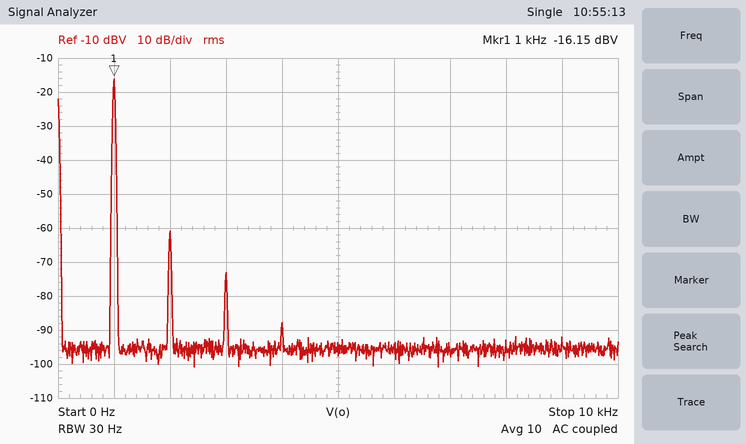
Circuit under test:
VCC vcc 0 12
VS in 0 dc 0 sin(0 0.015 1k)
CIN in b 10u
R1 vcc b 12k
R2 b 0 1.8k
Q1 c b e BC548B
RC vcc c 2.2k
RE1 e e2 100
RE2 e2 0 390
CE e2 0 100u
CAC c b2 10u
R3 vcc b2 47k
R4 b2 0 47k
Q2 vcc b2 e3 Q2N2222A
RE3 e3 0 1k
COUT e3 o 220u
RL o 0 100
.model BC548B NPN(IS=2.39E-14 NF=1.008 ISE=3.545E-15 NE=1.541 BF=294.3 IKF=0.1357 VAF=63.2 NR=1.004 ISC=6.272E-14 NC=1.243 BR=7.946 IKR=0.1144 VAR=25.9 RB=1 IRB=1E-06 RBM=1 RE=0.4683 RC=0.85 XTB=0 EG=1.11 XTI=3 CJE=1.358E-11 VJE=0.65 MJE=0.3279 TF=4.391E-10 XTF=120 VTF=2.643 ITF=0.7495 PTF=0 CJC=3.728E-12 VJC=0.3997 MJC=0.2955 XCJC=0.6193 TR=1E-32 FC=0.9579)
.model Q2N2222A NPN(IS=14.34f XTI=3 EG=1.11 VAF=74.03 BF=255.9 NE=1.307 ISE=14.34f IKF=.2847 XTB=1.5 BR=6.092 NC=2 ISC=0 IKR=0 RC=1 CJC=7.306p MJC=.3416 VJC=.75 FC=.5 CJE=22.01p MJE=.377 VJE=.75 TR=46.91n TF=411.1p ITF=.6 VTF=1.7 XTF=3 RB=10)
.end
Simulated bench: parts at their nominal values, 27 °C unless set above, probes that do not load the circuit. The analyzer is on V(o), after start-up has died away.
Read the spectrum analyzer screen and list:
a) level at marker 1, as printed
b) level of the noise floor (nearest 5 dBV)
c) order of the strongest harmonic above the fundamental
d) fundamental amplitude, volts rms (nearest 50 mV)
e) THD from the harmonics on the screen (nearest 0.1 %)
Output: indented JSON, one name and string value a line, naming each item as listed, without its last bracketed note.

{
  "level at marker 1, as printed": "-16.15 dBV",
  "level of the noise floor": "-95 dBV",
  "order of the strongest harmonic above the fundamental": "2",
  "fundamental amplitude, volts rms": "150 mV",
  "THD from the harmonics on the screen": "0.6 %"
}
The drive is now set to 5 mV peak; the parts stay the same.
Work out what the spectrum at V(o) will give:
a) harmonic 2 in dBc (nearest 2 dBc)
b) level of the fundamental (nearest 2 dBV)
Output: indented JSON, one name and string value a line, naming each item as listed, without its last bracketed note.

{
  "harmonic 2 in dBc": "-56 dBc",
  "level of the fundamental": "-26 dBV"
}
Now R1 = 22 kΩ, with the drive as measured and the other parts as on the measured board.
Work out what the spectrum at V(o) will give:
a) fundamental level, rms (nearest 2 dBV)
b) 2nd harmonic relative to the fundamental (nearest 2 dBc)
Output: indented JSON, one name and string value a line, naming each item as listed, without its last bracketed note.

{
  "fundamental level, rms": "-18 dBV",
  "2nd harmonic relative to the fundamental": "-42 dBc"
}
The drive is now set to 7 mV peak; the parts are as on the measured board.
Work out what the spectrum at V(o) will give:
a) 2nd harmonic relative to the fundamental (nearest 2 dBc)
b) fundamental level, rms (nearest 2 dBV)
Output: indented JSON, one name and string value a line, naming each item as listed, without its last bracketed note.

{
  "2nd harmonic relative to the fundamental": "-52 dBc",
  "fundamental level, rms": "-22 dBV"
}
